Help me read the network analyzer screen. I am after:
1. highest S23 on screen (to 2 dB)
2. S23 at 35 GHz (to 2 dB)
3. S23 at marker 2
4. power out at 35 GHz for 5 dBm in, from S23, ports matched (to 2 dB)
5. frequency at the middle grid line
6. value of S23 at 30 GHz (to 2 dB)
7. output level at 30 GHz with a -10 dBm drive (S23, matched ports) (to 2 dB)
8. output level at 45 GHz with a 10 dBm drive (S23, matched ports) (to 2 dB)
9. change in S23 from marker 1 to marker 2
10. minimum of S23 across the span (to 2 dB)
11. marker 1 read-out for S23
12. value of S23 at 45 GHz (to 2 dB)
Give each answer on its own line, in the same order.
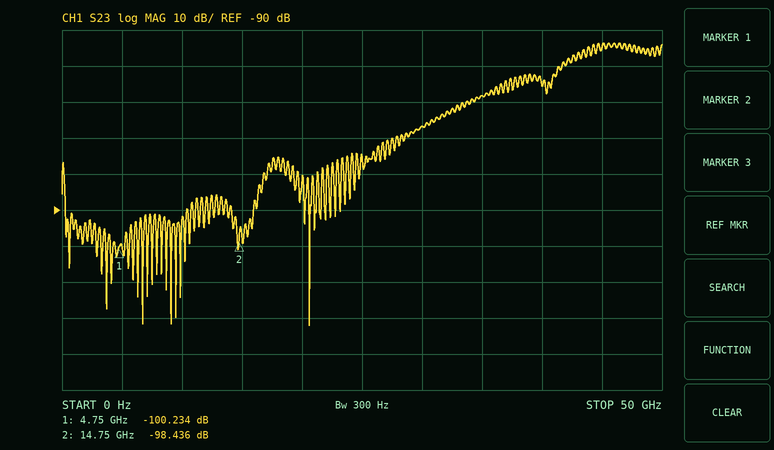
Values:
-44 dB
-58 dB
-98.436 dB
-54 dBm
25 GHz
-66 dB
-76 dBm
-34 dBm
1.798 dB
-122 dB
-100.234 dB
-44 dB
